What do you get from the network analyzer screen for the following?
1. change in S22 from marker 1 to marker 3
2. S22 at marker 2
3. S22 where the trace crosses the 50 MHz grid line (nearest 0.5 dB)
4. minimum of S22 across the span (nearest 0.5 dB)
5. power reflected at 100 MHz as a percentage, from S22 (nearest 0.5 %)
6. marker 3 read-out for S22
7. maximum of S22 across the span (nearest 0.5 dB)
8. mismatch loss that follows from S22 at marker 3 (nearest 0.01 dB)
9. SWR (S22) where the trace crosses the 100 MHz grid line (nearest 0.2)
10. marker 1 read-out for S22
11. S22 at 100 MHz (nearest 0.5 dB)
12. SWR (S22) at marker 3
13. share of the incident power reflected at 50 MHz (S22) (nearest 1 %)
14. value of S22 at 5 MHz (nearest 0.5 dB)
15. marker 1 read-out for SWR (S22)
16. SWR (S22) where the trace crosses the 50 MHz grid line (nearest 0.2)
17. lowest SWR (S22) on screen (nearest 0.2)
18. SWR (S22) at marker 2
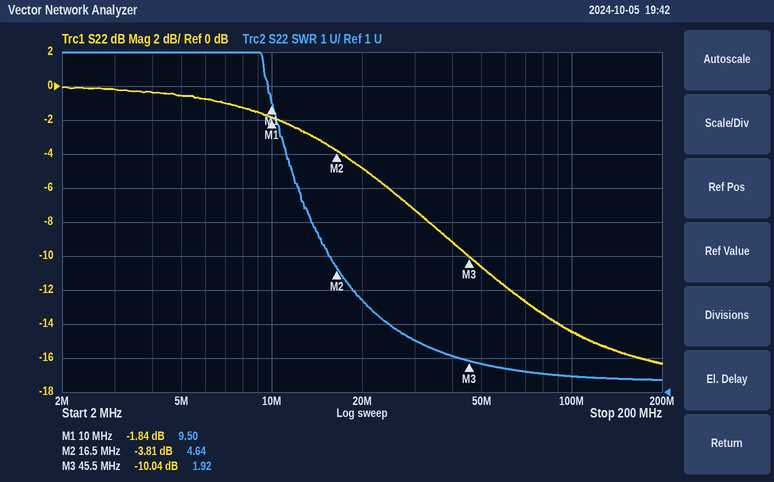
-8.20 dB
-3.81 dB
-10.5 dB
-16.5 dB
3.5 %
-10.04 dB
0.0 dB
0.45 dB
1.4
-1.84 dB
-14.5 dB
1.92
9 %
-0.5 dB
9.50
1.8
1.4
4.64
